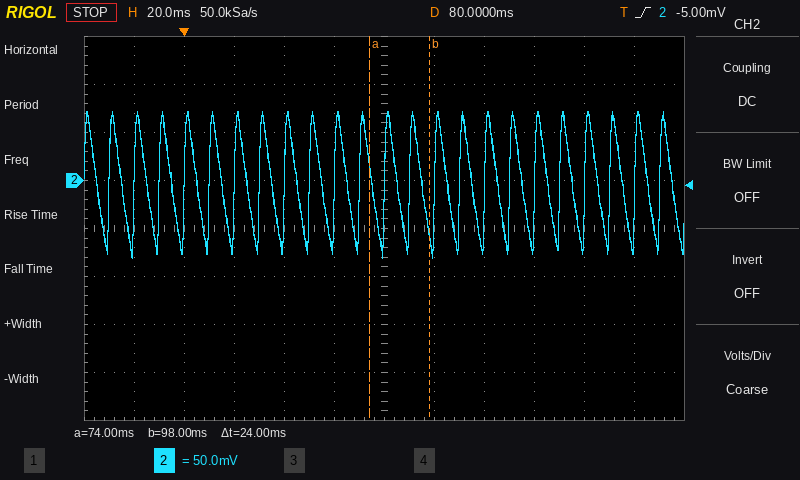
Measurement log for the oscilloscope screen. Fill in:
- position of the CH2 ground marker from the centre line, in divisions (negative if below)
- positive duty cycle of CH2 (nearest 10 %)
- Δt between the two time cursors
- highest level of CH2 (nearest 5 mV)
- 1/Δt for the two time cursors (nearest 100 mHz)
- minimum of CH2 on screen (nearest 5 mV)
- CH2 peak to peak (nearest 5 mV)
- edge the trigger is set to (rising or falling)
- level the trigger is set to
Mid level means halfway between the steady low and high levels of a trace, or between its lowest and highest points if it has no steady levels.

+1.0 div
50 %
24 ms
70 mV
41.7 Hz
-80 mV
150 mV
rising
-5.00 mV
